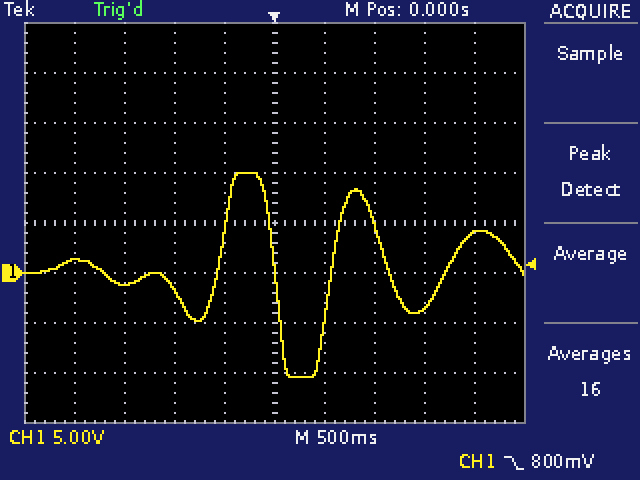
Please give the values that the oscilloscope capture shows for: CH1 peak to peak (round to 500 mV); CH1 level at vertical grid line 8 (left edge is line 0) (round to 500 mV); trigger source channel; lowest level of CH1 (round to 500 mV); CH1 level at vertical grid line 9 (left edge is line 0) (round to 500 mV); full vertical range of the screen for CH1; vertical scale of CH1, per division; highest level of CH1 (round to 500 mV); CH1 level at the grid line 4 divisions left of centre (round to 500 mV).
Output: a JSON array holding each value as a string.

["20.5 V", "-3.5 V", "CH1", "-10.5 V", "4.0 V", "40 V", "5 V", "10.0 V", "1.5 V"]
